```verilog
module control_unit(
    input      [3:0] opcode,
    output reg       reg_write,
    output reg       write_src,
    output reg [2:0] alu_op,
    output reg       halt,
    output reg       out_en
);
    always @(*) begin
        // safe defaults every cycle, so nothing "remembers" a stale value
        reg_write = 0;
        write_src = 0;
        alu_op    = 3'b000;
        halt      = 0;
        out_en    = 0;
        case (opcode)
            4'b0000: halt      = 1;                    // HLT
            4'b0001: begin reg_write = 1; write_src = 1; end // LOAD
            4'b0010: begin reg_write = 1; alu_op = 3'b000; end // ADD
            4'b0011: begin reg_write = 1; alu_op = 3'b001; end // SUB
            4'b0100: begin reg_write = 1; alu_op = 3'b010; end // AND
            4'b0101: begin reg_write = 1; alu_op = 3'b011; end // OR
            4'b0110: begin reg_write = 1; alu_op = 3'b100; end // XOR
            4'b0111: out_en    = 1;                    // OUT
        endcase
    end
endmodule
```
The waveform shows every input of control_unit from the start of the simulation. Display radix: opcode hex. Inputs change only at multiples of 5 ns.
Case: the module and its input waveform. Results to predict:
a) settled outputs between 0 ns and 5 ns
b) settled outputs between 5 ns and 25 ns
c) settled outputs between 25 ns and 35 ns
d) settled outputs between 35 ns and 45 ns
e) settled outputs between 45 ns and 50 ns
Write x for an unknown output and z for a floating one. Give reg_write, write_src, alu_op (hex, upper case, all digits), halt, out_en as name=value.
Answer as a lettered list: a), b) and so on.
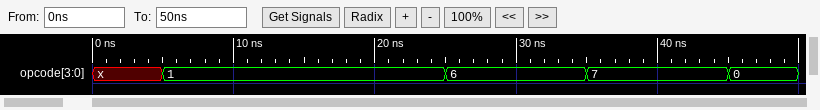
a) reg_write=x, write_src=x, alu_op=x, halt=x, out_en=x
b) reg_write=1, write_src=1, alu_op=0, halt=0, out_en=0
c) reg_write=1, write_src=0, alu_op=4, halt=0, out_en=0
d) reg_write=0, write_src=0, alu_op=0, halt=0, out_en=1
e) reg_write=0, write_src=0, alu_op=0, halt=1, out_en=0
